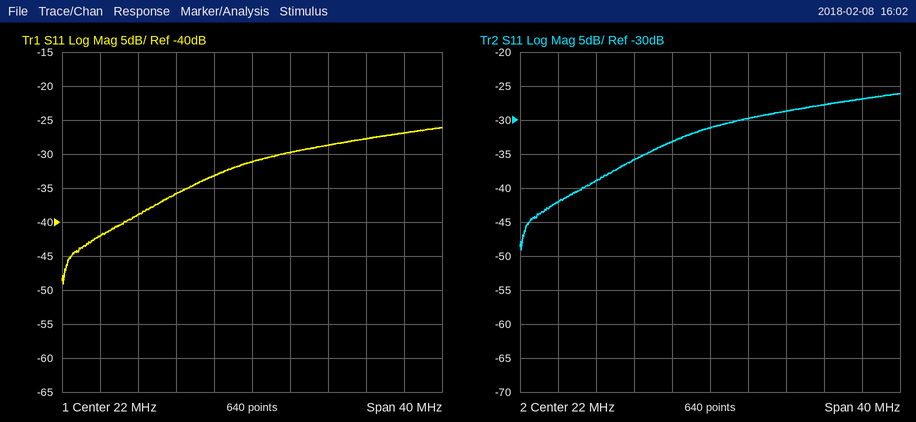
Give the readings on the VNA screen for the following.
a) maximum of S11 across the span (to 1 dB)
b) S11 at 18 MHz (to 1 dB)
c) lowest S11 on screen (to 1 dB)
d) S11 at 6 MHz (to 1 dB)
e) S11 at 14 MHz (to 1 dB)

-26 dB
-33 dB
-49 dB
-42 dB
-36 dB
